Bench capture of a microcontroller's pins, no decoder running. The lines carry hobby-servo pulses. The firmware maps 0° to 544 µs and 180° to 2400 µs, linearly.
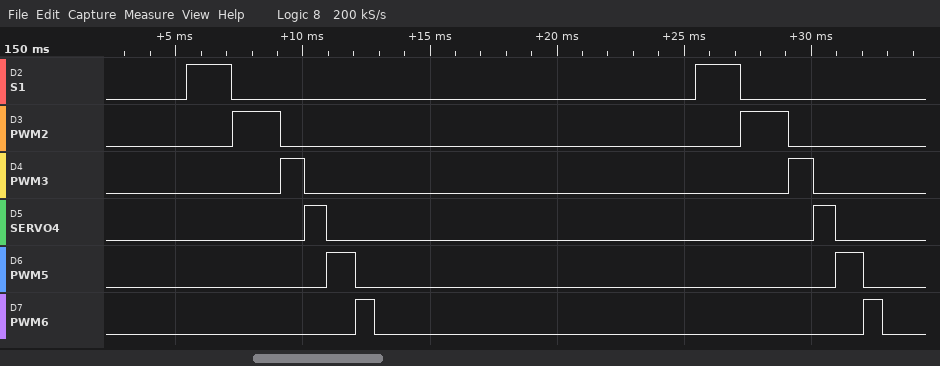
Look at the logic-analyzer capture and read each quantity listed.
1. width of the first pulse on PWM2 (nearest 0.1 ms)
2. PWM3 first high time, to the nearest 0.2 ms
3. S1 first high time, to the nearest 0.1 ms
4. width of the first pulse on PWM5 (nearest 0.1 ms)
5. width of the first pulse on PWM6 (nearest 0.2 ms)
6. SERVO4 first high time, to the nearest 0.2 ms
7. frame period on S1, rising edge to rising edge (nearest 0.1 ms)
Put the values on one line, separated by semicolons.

1.9 ms; 1.0 ms; 1.8 ms; 1.1 ms; 0.8 ms; 0.8 ms; 20.0 ms
